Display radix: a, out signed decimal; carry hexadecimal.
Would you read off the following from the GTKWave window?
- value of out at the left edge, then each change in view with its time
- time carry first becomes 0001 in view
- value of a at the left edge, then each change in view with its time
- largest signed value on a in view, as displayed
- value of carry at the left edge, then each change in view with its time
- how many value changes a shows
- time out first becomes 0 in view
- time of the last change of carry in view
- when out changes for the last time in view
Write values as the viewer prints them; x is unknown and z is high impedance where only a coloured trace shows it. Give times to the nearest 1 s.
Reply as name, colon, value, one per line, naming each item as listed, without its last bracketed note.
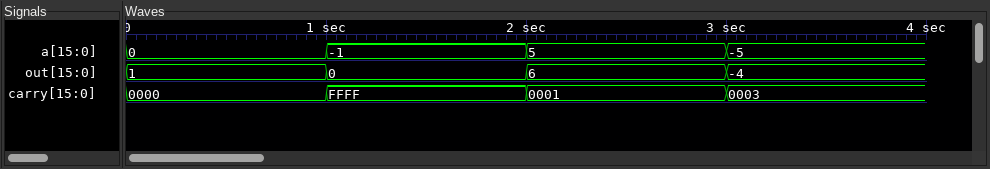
value of out at the left edge, then each change in view with its time: 1, 0 at 1 s, 6 at 2 s, -4 at 3 s
time carry first becomes 0001 in view: 2 s
value of a at the left edge, then each change in view with its time: 0, -1 at 1 s, 5 at 2 s, -5 at 3 s
largest signed value on a in view, as displayed: 5
value of carry at the left edge, then each change in view with its time: 0000, FFFF at 1 s, 0001 at 2 s, 0003 at 3 s
how many value changes a shows: 3
time out first becomes 0 in view: 1 s
time of the last change of carry in view: 3 s
when out changes for the last time in view: 3 s
